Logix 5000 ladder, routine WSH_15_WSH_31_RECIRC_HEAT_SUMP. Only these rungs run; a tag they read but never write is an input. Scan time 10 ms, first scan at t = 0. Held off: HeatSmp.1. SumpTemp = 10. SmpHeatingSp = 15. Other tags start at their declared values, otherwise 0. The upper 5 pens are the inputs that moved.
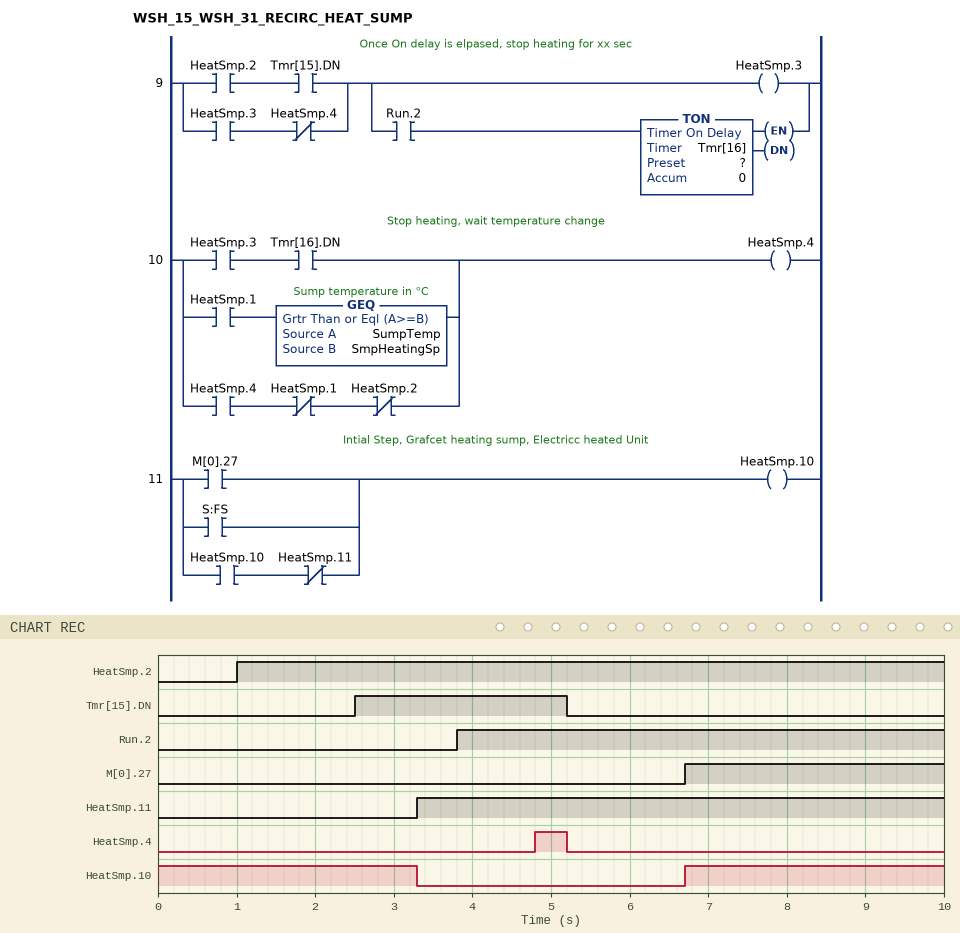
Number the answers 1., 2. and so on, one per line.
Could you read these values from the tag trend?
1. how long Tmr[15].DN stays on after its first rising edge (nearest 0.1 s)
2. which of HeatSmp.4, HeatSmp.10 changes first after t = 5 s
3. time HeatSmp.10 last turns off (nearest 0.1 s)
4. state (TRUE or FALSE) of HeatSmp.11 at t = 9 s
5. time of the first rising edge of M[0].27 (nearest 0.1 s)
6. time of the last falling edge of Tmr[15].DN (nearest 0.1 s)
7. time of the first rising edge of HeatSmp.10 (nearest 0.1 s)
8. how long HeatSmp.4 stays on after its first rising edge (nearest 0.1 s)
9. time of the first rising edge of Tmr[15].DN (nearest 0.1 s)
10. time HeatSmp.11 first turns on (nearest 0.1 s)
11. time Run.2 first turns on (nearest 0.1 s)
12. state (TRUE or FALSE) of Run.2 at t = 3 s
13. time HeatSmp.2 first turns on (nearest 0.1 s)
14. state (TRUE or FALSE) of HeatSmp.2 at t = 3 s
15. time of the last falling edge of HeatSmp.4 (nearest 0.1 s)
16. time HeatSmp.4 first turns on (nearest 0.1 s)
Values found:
1. 2.7 s
2. HeatSmp.4
3. 3.3 s
4. TRUE
5. 6.7 s
6. 5.2 s
7. 6.7 s
8. 0.4 s
9. 2.5 s
10. 3.3 s
11. 3.8 s
12. FALSE
13. 1.0 s
14. TRUE
15. 5.2 s
16. 4.8 s
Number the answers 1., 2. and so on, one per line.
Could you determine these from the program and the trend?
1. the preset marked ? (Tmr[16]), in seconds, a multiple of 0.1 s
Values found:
1. 1.0 s
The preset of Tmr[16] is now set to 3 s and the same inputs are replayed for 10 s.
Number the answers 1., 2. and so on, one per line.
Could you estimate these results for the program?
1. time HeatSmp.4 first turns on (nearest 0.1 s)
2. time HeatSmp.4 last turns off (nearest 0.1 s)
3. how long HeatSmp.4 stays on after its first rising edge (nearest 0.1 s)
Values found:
1. 6.8 s
2. 6.8 s
3. 0.0 s
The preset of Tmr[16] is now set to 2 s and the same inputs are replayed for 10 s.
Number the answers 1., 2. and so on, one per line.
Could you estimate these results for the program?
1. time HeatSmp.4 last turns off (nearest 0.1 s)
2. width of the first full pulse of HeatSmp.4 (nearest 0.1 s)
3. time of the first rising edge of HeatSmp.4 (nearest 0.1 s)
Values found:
1. 5.8 s
2. 0.0 s
3. 5.8 s
